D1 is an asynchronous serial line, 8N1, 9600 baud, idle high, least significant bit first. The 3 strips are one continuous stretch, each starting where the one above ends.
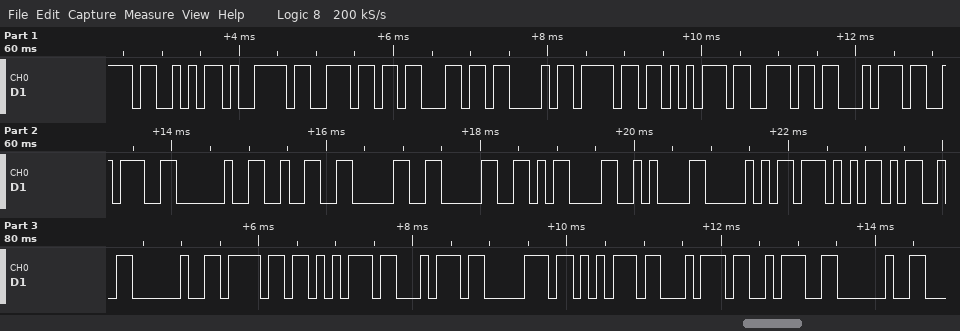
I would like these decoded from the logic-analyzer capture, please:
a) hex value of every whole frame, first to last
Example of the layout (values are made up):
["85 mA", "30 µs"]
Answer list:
["53 79 6E 63 43 6F 75 6E 74 3A 20 32 30 30 0D 0A 50 57 4D 20 6F 75 74 70 75 74 3A 20"]
